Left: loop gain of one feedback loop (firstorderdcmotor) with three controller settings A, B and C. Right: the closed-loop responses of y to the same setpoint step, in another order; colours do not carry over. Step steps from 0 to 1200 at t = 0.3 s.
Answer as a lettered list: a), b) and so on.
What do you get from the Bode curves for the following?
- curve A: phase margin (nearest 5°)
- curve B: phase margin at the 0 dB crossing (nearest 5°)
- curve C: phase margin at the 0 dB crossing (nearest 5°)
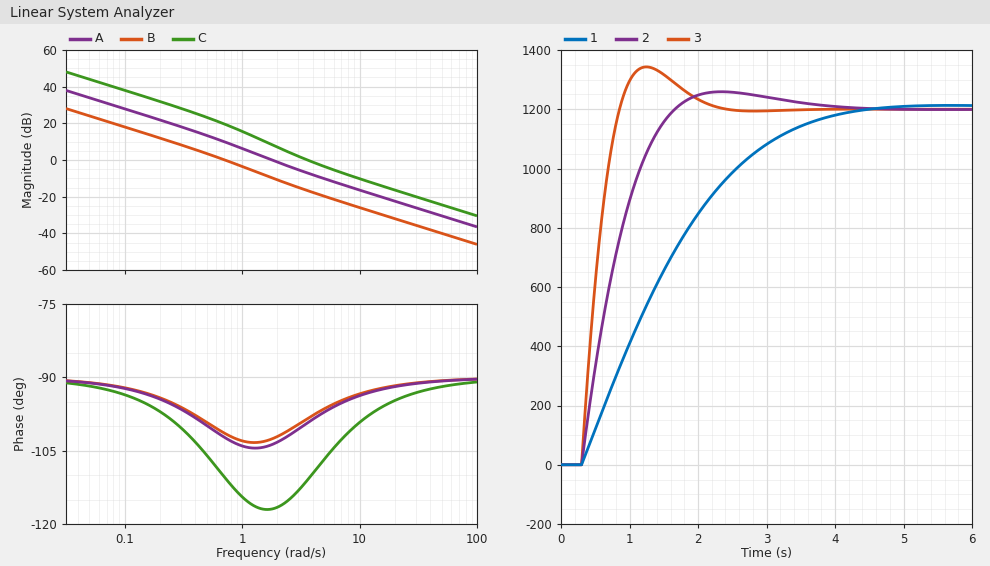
a) 75°
b) 80°
c) 70°
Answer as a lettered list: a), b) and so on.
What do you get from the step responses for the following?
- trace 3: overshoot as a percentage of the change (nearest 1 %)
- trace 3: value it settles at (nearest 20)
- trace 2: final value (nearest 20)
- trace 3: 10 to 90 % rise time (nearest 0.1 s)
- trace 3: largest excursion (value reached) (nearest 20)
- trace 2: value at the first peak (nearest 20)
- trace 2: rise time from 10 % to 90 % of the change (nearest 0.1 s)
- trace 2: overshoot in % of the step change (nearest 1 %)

a) 12 %
b) 1200
c) 1200
d) 0.4 s
e) 1340
f) 1260
g) 0.9 s
h) 5 %
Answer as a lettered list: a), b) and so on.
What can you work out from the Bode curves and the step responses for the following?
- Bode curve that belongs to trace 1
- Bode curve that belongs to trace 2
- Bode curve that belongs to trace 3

a) B
b) A
c) C
